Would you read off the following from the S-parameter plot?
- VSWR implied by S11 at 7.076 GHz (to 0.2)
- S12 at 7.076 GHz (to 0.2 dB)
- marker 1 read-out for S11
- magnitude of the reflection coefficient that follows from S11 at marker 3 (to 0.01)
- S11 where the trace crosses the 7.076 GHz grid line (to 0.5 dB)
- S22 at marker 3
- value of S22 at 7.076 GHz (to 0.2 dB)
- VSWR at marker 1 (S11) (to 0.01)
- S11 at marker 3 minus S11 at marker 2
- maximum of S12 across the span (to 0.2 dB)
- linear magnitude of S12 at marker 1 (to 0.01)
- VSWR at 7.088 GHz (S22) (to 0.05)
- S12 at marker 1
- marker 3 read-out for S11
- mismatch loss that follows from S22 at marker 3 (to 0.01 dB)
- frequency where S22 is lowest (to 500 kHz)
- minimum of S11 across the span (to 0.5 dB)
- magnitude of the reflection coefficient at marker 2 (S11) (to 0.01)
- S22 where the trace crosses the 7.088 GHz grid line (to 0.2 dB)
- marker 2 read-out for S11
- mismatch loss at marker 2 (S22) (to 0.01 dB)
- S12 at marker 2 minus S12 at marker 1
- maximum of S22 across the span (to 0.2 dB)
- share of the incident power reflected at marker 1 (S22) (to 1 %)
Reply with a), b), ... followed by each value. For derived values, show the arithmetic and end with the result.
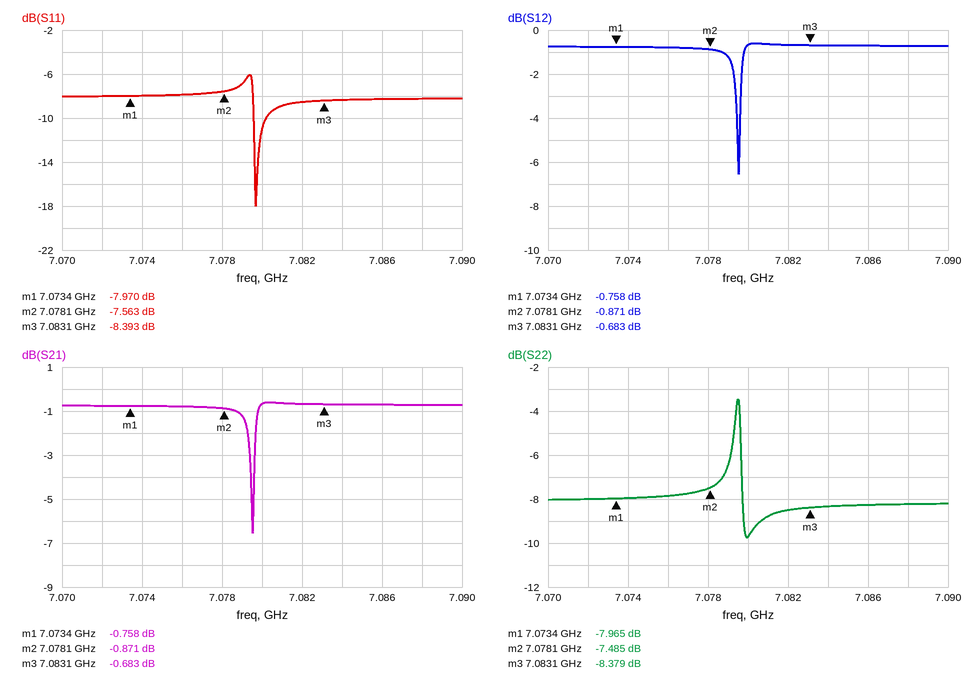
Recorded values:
a) |Γ| = 10^(-8/20) = 0.3981; VSWR = (1 + 0.3981)/(1 − 0.3981) ≈ 2.32, so 2.4 to the nearest 0.2
b) -0.8 dB
c) -7.970 dB
d) 10^(-8.393/20) ≈ 0.38
e) -8.0 dB
f) -8.379 dB
g) -7.8 dB
h) (1 + 0.3995)/(1 − 0.3995) ≈ 2.33
i) -8.393 − (-7.563) = -0.830 dB
j) -0.6 dB
k) 10^(-0.758/20) ≈ 0.92
l) |Γ| = 10^(-8.2/20) = 0.3890; VSWR = (1 + 0.3890)/(1 − 0.3890) ≈ 2.27, so 2.25 to the nearest 0.05
m) -0.758 dB
n) -8.393 dB
o) −10 log10(1 − 10^(-8.379/10)) ≈ 0.68 dB
p) 7.0800 GHz
q) -18.0 dB
r) 10^(-7.563/20) ≈ 0.42
s) -8.2 dB
t) -7.563 dB
u) −10 log10(1 − 10^(-7.485/10)) ≈ 0.85 dB
v) -0.871 − (-0.758) = -0.113 dB
w) -3.4 dB
x) 10^(-7.965/10) ≈ 16 %
